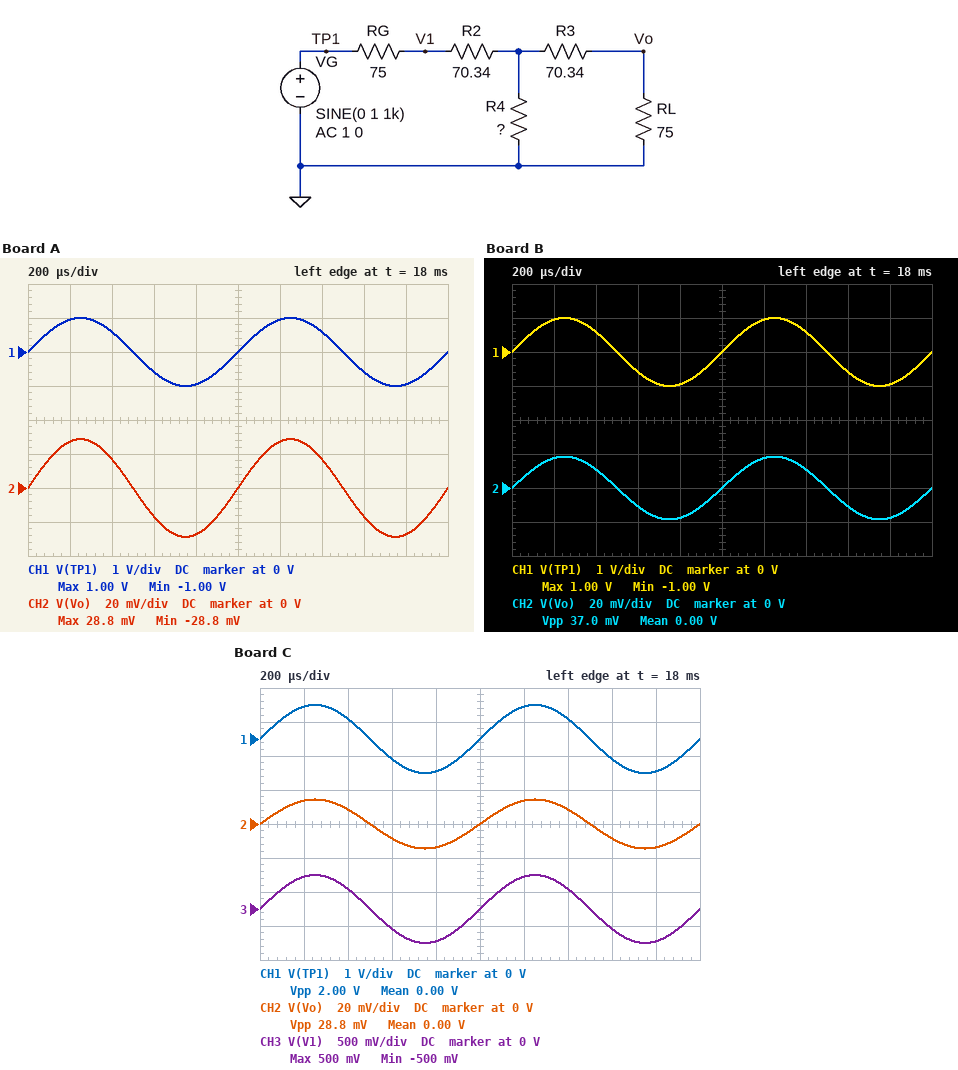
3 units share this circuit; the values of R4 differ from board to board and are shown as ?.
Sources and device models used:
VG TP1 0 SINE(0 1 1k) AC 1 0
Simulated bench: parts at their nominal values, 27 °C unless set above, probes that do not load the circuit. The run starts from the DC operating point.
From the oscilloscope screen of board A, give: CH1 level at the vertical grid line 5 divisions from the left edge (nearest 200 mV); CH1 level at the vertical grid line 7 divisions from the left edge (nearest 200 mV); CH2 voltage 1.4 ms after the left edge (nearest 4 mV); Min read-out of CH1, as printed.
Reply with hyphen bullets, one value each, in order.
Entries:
- 0 V
- 600 mV
- 16 mV
- -1.00 V
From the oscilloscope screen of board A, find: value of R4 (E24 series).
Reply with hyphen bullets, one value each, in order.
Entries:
- 9.1 Ω
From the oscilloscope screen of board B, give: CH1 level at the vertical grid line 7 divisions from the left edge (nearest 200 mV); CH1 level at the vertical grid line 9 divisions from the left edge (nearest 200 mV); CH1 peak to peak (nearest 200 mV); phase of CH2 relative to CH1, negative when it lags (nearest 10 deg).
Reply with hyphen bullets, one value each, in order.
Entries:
- 600 mV
- -1.0 V
- 2.0 V
- 0 deg
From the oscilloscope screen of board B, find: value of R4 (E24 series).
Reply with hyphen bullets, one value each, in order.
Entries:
- 5.6 Ω
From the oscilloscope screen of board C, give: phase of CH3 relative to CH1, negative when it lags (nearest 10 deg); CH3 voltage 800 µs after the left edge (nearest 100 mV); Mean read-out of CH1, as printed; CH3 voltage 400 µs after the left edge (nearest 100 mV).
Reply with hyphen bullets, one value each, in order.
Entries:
- 0 deg
- -500 mV
- 0.00 V
- 300 mV
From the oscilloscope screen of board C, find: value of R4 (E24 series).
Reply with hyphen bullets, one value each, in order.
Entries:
- 4.3 Ω
